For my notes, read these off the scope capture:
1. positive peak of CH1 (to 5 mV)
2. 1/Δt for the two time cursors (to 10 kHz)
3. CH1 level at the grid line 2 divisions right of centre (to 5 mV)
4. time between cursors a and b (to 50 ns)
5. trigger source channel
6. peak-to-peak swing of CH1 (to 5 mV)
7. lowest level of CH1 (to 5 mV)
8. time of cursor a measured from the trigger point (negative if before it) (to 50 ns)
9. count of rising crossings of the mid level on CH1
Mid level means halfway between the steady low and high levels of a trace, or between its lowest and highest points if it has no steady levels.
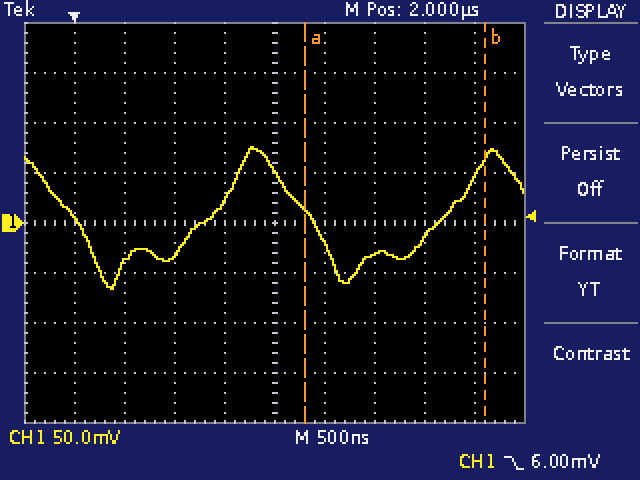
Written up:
75 mV
560 kHz
-30 mV
1.80 µs
CH1
140 mV
-65 mV
+2.30 µs
2
